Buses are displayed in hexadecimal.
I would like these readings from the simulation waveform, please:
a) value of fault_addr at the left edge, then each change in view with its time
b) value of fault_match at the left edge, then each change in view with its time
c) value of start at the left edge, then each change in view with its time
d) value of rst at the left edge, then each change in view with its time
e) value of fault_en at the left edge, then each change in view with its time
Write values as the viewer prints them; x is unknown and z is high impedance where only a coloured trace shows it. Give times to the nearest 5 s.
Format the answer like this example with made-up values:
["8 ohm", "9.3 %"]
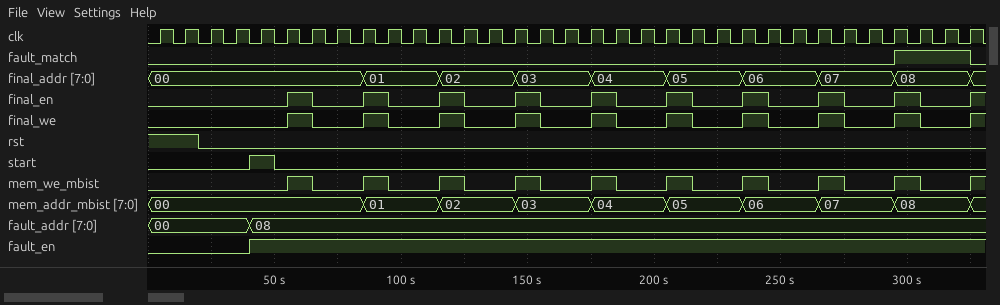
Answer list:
["00, 08 at 40 s", "0, 1 at 295 s, 0 at 325 s", "0, 1 at 40 s, 0 at 50 s", "1, 0 at 20 s", "0, 1 at 40 s"]
